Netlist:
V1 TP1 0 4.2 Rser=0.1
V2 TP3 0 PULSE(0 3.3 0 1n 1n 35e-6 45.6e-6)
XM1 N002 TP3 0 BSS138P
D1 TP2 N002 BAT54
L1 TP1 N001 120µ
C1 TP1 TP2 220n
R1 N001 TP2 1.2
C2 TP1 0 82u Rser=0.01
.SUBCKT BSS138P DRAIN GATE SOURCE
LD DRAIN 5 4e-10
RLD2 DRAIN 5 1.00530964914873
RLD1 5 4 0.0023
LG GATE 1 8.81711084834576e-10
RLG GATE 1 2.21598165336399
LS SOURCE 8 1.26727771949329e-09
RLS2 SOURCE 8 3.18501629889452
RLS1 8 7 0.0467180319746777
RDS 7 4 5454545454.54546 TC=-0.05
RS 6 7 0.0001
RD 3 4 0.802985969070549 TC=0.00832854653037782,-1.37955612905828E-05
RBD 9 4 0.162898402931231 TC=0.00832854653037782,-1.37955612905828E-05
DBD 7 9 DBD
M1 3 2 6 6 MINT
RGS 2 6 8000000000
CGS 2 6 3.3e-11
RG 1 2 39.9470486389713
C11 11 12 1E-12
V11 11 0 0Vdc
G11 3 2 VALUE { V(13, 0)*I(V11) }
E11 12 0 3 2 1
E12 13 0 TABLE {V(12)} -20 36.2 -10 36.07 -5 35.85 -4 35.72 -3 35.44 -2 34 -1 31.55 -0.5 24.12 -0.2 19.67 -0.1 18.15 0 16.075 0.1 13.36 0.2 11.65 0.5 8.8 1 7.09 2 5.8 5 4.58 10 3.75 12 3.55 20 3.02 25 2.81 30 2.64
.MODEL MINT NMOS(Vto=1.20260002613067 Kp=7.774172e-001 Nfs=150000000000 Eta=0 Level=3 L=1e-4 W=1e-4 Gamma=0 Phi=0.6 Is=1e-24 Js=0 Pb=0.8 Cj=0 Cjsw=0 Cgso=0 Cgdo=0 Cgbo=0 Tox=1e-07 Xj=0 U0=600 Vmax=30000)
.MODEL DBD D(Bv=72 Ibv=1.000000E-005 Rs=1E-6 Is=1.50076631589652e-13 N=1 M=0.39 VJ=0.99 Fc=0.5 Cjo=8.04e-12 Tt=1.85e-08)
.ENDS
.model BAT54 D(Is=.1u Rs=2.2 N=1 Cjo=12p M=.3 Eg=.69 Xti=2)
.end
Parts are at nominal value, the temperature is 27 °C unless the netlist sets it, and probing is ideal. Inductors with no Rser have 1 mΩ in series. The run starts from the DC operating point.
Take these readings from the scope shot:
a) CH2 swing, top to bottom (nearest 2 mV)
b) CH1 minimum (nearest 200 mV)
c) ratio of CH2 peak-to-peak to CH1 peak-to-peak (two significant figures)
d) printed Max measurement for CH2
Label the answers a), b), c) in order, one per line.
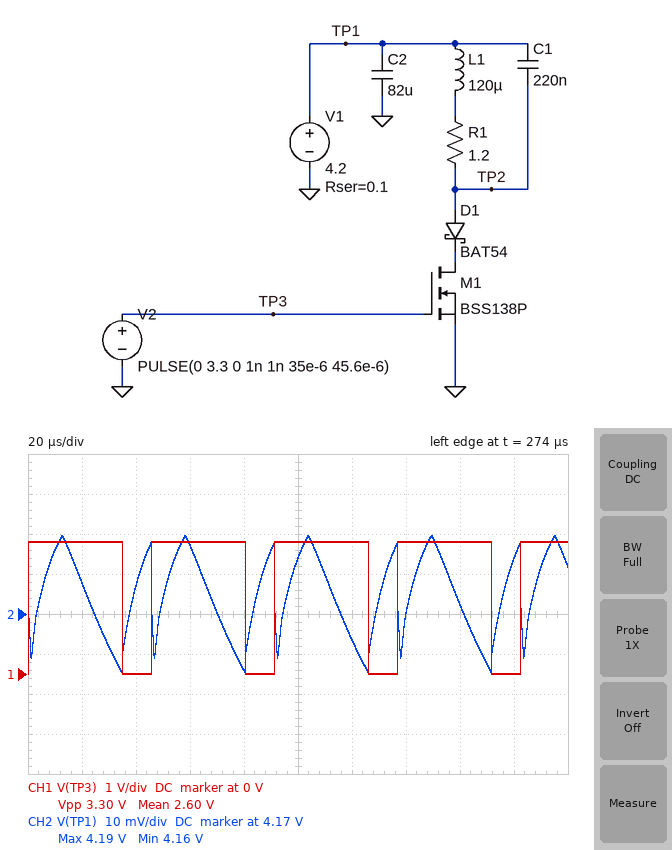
a) 34 mV
b) 0 V
c) 0.010
d) 4.19 V
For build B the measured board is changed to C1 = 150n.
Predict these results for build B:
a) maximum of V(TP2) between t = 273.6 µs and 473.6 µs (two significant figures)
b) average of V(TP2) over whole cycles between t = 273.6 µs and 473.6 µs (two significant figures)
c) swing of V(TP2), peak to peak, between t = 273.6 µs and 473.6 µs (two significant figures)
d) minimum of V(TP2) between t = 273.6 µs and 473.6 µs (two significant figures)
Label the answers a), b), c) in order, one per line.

a) 22 V
b) 3.8 V
c) 32 V
d) -10 V
